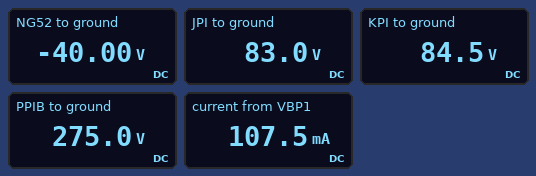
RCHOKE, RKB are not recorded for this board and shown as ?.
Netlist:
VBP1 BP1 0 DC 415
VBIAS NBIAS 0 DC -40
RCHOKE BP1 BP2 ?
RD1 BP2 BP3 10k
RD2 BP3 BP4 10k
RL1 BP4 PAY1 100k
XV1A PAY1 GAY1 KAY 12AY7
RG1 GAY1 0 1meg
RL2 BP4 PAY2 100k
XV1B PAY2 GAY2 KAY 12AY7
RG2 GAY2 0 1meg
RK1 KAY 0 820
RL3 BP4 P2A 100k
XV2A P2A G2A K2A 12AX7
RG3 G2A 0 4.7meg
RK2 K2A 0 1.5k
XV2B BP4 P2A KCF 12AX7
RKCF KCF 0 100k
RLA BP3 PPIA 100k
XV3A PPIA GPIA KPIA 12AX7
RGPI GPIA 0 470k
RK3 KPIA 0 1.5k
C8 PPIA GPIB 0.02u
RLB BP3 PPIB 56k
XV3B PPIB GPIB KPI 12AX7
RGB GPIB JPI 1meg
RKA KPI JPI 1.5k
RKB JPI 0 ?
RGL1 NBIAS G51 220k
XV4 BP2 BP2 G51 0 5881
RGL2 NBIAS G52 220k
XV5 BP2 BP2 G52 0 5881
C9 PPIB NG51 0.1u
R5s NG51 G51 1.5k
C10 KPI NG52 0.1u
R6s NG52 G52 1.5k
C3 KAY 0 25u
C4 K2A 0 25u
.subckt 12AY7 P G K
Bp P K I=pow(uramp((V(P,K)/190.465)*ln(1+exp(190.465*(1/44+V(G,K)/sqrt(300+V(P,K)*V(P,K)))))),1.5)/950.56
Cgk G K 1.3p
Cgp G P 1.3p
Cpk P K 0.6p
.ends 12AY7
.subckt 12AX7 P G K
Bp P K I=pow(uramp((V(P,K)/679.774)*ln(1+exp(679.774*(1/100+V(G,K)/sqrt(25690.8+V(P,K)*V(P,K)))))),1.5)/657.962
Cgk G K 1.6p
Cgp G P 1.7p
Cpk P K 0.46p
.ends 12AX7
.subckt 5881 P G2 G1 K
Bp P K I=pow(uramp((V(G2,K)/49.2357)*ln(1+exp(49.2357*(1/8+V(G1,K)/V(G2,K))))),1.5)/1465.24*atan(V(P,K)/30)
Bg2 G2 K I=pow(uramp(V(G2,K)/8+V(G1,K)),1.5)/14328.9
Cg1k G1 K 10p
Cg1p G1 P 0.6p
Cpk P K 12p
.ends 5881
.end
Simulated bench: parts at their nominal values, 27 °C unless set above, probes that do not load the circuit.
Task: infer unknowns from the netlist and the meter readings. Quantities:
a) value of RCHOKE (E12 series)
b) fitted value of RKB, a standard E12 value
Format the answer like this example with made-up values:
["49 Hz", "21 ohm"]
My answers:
["68 Ω", "82 kΩ"]
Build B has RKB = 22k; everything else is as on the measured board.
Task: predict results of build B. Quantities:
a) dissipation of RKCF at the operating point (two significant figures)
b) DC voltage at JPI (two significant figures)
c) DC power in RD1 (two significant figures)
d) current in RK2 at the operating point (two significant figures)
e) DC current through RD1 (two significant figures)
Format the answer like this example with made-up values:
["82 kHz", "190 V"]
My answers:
["320 mW", "27 V", "600 mW", "960 µA", "7.8 mA"]
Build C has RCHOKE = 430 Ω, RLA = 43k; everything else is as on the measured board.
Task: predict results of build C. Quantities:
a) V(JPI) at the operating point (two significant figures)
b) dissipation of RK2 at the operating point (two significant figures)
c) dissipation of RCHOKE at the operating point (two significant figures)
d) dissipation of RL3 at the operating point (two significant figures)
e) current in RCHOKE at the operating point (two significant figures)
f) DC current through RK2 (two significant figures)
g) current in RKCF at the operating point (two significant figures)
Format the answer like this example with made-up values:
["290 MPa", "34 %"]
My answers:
["78 V", "1.2 mW", "2.5 W", "81 mW", "77 mA", "900 µA", "1.7 mA"]
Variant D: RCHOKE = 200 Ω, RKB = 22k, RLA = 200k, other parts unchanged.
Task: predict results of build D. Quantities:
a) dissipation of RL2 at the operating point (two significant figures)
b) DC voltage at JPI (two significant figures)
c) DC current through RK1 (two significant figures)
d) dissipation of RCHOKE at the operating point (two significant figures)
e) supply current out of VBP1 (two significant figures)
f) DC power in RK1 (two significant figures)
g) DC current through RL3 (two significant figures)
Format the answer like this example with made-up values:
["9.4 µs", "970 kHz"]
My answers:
["170 mW", "26 V", "2.6 mA", "1.7 W", "93 mA", "5.6 mW", "940 µA"]
